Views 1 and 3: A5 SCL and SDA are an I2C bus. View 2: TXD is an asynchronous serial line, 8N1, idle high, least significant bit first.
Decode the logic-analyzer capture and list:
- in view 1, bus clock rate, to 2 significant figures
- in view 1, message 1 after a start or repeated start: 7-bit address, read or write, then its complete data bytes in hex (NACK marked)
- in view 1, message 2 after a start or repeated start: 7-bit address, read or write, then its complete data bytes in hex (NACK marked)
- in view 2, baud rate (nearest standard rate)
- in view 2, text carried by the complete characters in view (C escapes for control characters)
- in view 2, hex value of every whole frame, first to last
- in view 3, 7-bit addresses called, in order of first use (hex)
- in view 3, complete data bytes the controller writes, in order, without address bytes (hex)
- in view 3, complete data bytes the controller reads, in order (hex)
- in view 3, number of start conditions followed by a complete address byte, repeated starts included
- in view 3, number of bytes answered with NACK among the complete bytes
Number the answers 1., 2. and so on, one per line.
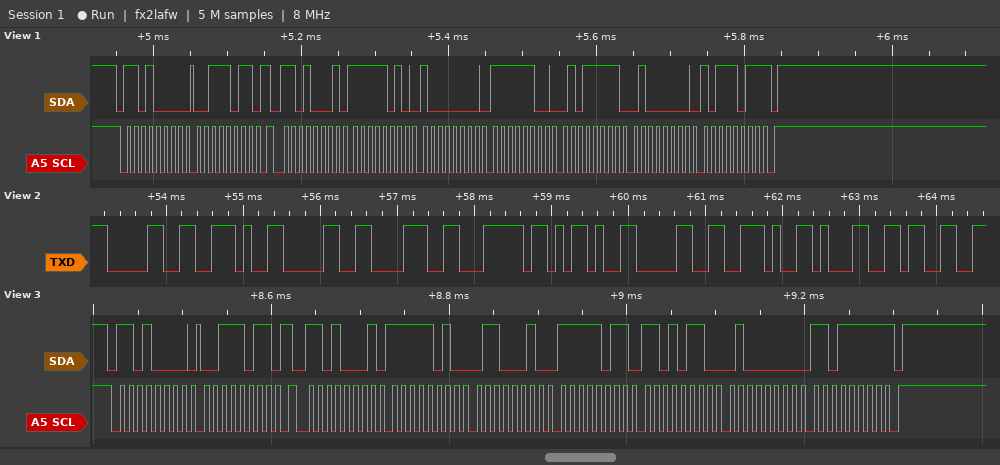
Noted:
1. 100 kHz
2. 0x68 write: 3B
3. 0x68 read: FA 80 FC 5F 40 BB NACK
4. 9600 baud
5. "0.08|-0.13"
6. 30 2E 30 38 7C 2D 30 2E 31 33
7. 0x68
8. 3B
9. FA 62 FB D6 40 DF
10. 2
11. 1
